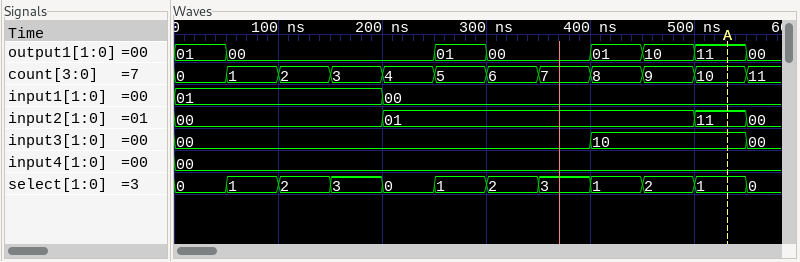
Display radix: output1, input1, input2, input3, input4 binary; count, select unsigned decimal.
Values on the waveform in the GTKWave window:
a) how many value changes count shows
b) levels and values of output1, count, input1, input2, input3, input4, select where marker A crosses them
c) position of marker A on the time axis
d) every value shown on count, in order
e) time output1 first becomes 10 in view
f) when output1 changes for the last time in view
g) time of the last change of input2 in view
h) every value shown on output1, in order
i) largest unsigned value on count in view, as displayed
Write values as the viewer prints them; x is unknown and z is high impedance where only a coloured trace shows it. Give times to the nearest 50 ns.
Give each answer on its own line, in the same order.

11
output1=11, count=10, input1=00, input2=11, input3=10, input4=00, select=1
550 ns
0, 1, 2, 3, 4, 5, 6, 7, 8, 9, 10, 11
450 ns
550 ns
550 ns
01, 00, 01, 00, 01, 10, 11, 00
11
